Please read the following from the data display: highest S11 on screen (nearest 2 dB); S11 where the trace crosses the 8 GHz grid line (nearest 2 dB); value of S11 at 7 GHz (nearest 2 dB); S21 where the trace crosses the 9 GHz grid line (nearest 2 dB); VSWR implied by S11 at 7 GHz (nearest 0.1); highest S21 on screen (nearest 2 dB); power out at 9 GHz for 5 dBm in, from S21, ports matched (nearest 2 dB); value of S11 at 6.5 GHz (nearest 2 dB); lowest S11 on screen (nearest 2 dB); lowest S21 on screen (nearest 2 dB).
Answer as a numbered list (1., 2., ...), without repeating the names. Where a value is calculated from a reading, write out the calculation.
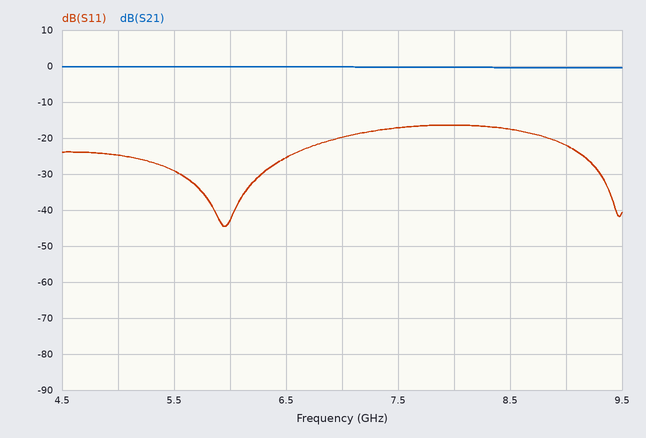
1. -16 dB
2. -16 dB
3. -20 dB
4. 0 dB
5. |Γ| = 10^(-20/20) = 0.1000; VSWR = (1 + 0.1000)/(1 − 0.1000) ≈ 1.2
6. 0 dB
7. 5 dBm + (0 dB) = 4 dBm
8. -26 dB
9. -44 dB
10. 0 dB
